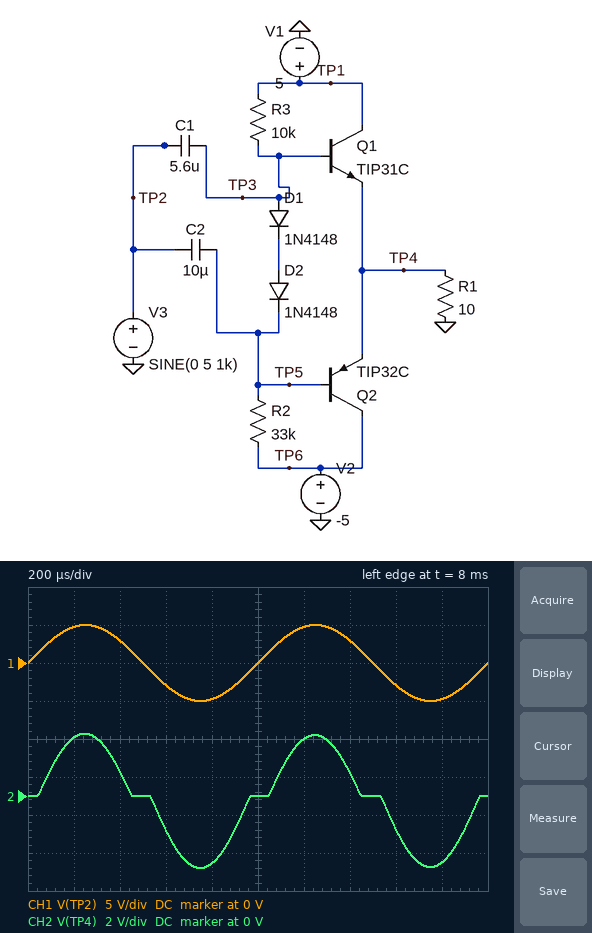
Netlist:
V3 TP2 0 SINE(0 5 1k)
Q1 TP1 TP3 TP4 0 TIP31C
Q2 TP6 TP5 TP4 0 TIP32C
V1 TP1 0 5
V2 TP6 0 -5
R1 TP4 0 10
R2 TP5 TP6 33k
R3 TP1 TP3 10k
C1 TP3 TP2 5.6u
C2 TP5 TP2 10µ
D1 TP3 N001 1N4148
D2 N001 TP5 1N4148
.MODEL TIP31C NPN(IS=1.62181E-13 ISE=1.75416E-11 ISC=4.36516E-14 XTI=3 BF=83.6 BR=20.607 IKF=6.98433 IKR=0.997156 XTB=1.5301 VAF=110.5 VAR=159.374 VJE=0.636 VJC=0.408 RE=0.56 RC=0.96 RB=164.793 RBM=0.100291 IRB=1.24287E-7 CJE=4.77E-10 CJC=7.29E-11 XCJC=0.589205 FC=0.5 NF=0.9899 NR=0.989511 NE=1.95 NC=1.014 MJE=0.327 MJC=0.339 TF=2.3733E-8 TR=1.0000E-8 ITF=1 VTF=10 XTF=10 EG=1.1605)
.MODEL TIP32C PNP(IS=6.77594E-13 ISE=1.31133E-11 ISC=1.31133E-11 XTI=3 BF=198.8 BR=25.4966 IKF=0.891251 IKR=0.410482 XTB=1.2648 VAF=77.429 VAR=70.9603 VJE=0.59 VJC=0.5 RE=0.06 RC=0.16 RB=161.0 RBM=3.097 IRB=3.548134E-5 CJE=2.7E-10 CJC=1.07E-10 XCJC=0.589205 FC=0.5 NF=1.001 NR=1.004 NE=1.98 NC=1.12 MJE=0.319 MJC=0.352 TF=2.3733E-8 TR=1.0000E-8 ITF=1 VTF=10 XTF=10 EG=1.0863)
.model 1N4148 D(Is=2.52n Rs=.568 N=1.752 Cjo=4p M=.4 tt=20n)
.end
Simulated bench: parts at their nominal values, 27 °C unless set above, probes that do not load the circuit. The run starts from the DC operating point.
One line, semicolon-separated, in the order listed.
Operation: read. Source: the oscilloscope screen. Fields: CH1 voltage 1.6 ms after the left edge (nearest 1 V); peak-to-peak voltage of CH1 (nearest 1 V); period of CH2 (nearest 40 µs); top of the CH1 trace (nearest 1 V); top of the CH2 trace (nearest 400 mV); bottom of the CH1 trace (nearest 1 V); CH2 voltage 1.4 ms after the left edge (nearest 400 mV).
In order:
-3 V; 10 V; 1.00 ms; 5 V; 3.2 V; -5 V; 1.2 V
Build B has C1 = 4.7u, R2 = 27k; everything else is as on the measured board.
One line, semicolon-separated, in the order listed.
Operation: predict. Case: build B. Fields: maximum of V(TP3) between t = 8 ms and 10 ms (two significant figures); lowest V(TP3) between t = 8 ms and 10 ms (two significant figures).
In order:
4.1 V; -6.0 V
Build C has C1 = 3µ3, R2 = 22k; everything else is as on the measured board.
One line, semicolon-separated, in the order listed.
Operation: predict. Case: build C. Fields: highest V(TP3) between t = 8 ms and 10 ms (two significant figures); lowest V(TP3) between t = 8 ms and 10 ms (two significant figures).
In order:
3.8 V; -6.3 V
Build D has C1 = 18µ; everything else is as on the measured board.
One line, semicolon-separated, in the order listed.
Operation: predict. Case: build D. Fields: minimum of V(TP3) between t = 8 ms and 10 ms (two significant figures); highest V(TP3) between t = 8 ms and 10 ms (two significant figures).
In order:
-5.2 V; 4.9 V
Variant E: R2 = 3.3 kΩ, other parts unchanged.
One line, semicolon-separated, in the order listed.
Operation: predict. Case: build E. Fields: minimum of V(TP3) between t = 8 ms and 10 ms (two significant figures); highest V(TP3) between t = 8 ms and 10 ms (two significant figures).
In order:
-6.2 V; 3.8 V
